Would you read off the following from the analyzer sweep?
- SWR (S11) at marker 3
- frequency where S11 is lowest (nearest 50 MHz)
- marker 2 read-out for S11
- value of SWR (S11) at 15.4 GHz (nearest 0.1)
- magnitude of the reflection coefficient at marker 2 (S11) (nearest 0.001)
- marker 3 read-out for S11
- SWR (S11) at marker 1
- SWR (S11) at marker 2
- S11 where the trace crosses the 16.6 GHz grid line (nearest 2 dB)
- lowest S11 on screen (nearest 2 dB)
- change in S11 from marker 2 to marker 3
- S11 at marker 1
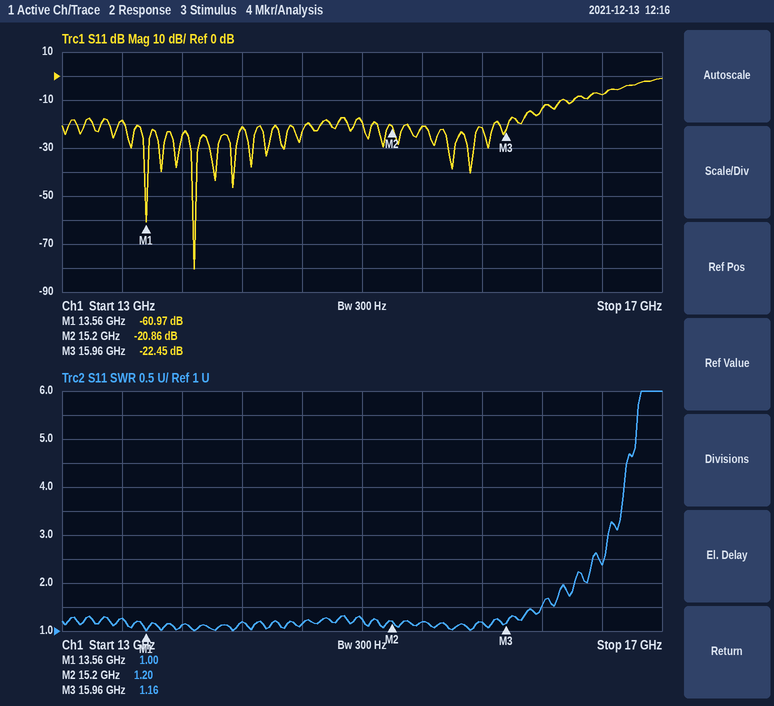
1.16
13.90 GHz
-20.86 dB
1.2
0.091
-22.45 dB
1.00
1.20
-8 dB
-80 dB
-1.59 dB
-60.97 dB
